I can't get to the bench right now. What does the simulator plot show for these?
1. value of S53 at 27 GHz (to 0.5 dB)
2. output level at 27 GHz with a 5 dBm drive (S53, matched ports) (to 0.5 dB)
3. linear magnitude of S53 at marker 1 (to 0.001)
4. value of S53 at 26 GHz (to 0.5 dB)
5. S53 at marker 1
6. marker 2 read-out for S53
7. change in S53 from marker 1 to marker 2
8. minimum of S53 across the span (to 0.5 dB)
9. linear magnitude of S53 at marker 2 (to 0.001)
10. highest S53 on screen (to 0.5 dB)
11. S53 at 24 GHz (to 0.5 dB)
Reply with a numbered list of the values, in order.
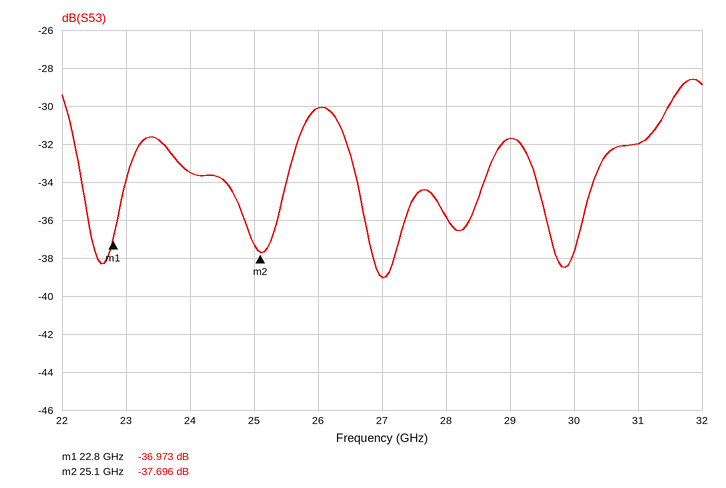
1. -39.0 dB
2. -34.0 dBm
3. 0.014
4. -30.0 dB
5. -36.973 dB
6. -37.696 dB
7. -0.723 dB
8. -39.0 dB
9. 0.013
10. -28.5 dB
11. -33.5 dB
